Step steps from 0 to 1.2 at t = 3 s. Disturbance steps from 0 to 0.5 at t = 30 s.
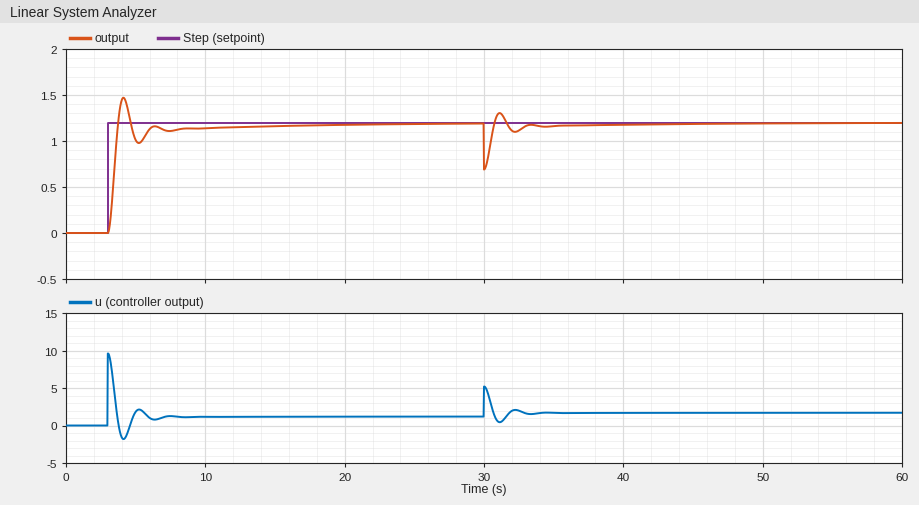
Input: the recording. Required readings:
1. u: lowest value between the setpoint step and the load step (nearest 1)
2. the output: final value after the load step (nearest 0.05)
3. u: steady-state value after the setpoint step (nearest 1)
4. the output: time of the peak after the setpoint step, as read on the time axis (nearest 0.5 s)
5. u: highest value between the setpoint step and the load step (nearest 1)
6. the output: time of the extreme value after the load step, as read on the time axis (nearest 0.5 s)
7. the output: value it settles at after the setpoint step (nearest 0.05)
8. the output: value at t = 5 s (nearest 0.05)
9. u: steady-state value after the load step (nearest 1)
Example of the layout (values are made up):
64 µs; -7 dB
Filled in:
-2; 1.20; 1; 4.0 s; 10; 30.0 s; 1.20; 1.00; 2
